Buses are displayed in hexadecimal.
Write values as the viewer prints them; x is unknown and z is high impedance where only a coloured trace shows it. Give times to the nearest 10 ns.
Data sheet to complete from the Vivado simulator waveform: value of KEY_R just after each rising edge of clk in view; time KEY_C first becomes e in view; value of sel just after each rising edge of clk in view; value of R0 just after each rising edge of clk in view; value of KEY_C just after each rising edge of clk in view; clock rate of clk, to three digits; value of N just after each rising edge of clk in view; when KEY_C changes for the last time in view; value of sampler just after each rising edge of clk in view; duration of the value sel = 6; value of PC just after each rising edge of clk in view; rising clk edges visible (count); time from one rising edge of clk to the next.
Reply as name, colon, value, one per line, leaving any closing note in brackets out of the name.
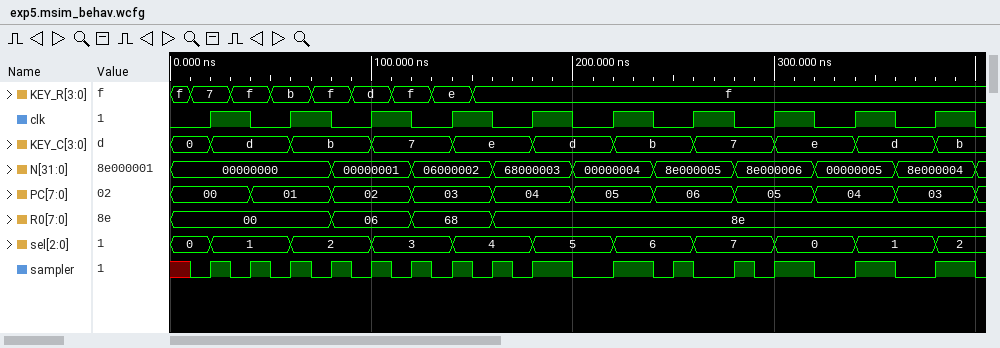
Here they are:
value of KEY_R just after each rising edge of clk in view: 7, b, d, e, f, f, f, f, f, f
time KEY_C first becomes e in view: 140 ns
value of sel just after each rising edge of clk in view: 1, 2, 3, 4, 5, 6, 7, 0, 1, 2
value of R0 just after each rising edge of clk in view: 00, 00, 06, 68, 8e, 8e, 8e, 8e, 8e, 8e
value of KEY_C just after each rising edge of clk in view: d, b, 7, e, d, b, 7, e, d, b
clock rate of clk, to three digits: 25.0 MHz
value of N just after each rising edge of clk in view: 00000000, 00000000, 00000001, 06000002, 68000003, 00000004, 8e000005, 8e000006, 00000005, 8e000004
when KEY_C changes for the last time in view: 380 ns
value of sampler just after each rising edge of clk in view: 1 1 1 1 1 1 0 1 1 1
duration of the value sel = 6: 40 ns
value of PC just after each rising edge of clk in view: 00, 01, 02, 03, 04, 05, 06, 05, 04, 03
rising clk edges visible: 10
time from one rising edge of clk to the next: 40 ns
